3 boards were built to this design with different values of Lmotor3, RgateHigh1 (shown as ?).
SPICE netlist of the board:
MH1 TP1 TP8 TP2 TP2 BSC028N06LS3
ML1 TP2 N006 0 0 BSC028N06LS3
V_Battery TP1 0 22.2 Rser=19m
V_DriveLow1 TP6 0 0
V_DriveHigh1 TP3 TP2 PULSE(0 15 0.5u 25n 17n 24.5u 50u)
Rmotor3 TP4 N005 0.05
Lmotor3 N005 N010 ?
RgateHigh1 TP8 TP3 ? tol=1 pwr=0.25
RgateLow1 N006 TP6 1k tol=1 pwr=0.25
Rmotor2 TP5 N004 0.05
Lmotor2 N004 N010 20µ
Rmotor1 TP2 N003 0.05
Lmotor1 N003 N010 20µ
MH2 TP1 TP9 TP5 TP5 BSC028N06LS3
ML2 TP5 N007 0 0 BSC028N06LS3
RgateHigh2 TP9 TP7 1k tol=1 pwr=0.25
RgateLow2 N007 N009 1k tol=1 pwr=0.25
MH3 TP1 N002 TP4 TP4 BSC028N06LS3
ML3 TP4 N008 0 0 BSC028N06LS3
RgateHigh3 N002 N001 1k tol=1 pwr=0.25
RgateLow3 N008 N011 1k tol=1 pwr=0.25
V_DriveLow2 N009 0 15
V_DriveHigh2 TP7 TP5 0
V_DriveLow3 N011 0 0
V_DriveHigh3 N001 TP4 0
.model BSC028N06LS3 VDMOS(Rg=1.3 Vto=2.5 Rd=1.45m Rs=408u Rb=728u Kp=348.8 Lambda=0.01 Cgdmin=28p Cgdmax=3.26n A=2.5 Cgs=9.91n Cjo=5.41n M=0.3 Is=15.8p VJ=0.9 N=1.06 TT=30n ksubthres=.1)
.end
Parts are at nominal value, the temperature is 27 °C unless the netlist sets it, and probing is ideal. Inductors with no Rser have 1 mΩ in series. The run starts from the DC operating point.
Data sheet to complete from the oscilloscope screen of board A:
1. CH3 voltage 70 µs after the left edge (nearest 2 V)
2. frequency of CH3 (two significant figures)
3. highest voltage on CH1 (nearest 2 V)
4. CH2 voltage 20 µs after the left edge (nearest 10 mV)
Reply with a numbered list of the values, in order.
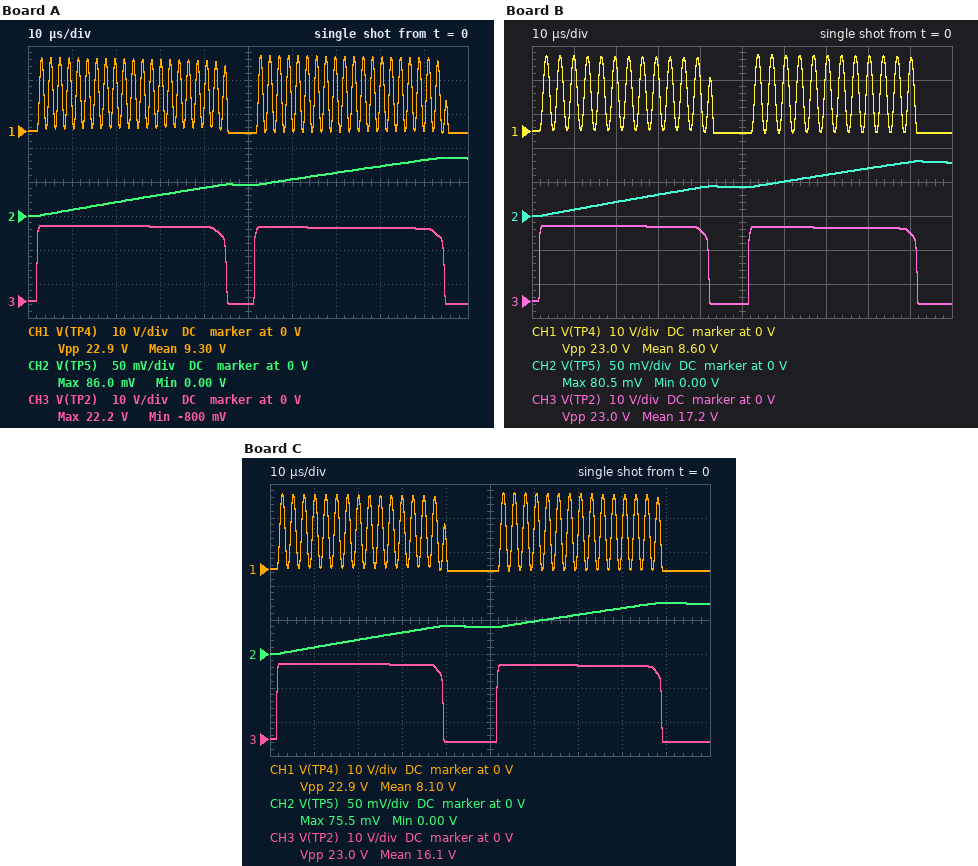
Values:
1. 22 V
2. 20 kHz
3. 22 V
4. 20 mV
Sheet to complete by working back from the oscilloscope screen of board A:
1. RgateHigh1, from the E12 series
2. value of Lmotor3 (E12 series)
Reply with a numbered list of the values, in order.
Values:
1. 820 Ω
2. 10 µH
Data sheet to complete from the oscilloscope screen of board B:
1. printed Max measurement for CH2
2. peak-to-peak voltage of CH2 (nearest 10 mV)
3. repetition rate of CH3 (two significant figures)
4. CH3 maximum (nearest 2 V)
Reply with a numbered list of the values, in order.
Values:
1. 80.5 mV
2. 80 mV
3. 20 kHz
4. 22 V
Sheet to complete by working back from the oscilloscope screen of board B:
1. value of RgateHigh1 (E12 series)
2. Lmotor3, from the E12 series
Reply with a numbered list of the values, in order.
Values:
1. 680 Ω
2. 39 µH
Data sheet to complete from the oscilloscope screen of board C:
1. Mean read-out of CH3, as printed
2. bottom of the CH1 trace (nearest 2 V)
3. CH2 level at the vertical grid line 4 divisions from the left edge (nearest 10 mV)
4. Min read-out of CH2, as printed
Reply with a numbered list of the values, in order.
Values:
1. 16.1 V
2. 0 V
3. 40 mV
4. 0.00 V
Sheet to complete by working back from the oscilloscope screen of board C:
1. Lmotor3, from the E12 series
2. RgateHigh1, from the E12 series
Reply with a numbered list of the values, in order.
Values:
1. 18 µH
2. 560 Ω
